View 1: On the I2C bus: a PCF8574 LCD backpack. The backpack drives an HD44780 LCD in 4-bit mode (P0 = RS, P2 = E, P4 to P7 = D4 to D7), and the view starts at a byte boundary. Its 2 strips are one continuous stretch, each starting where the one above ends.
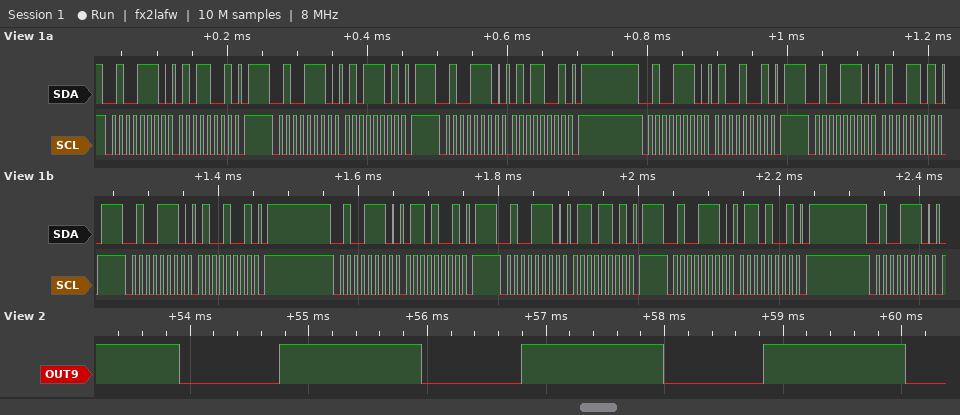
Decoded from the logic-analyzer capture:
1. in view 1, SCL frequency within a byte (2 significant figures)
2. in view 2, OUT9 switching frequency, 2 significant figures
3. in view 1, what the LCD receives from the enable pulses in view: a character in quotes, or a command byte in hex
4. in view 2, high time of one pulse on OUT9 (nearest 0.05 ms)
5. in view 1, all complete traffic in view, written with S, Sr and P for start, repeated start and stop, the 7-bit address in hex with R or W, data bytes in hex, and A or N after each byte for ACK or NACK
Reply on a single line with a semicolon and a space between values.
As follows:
100 kHz; 490 Hz; 'T'; 1.20 ms; S 27W A 59 A P S 27W A 5D A P S 27W A 59 A P S 27W A 49 A P S 27W A 4D A P S 27W A 49 A P S 27W A 69 A P S 27W A 6D A P S 27W A 69 A P S 27W A
